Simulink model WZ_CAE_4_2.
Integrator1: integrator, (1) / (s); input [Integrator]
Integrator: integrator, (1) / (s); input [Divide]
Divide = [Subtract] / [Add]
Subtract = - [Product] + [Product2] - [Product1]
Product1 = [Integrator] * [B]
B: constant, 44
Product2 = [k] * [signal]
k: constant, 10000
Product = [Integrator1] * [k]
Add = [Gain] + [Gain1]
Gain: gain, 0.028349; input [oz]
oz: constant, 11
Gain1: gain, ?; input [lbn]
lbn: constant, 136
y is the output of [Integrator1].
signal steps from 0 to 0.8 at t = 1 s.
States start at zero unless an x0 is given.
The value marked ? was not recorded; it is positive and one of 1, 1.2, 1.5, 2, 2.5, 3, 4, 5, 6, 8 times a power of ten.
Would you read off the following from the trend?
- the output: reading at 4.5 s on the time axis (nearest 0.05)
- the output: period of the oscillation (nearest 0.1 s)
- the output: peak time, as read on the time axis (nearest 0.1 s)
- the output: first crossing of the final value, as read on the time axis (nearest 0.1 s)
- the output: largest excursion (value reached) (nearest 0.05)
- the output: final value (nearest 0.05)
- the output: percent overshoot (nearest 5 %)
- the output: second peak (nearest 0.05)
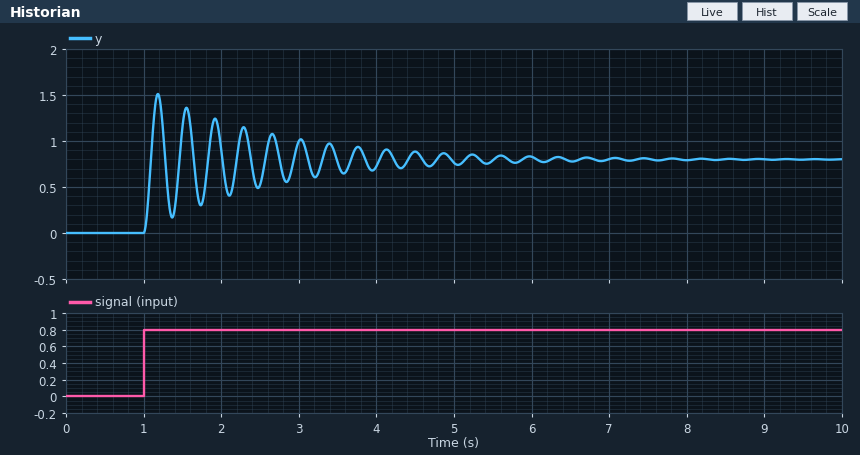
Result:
0.90
0.4 s
1.2 s
1.1 s
1.50
0.80
90 %
1.35
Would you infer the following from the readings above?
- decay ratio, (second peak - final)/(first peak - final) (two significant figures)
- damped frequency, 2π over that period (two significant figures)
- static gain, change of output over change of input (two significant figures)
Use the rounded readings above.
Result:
0.79
16 rad/s
1.0
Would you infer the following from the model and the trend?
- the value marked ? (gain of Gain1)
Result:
0.25
